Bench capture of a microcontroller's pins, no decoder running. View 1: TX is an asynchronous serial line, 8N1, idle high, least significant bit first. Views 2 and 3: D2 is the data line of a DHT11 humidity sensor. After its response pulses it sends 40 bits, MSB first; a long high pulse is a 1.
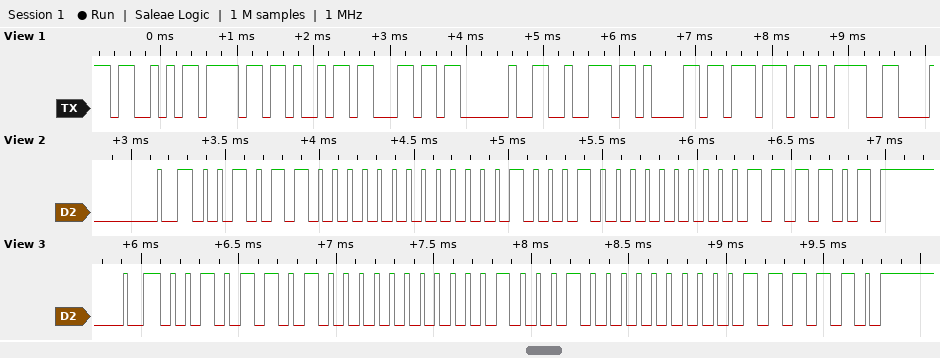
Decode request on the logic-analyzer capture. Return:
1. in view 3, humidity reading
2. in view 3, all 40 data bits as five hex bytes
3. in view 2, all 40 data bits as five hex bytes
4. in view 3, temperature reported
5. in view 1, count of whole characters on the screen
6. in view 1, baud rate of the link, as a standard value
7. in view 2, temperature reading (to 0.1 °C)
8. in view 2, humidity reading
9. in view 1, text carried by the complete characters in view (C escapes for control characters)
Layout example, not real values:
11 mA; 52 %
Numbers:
45 %; 2D 00 11 00 3E; 2C 00 11 00 3D; 17.0 °C; 9; 9600 baud; 17.0 °C; 44 %; "Soil raw="
